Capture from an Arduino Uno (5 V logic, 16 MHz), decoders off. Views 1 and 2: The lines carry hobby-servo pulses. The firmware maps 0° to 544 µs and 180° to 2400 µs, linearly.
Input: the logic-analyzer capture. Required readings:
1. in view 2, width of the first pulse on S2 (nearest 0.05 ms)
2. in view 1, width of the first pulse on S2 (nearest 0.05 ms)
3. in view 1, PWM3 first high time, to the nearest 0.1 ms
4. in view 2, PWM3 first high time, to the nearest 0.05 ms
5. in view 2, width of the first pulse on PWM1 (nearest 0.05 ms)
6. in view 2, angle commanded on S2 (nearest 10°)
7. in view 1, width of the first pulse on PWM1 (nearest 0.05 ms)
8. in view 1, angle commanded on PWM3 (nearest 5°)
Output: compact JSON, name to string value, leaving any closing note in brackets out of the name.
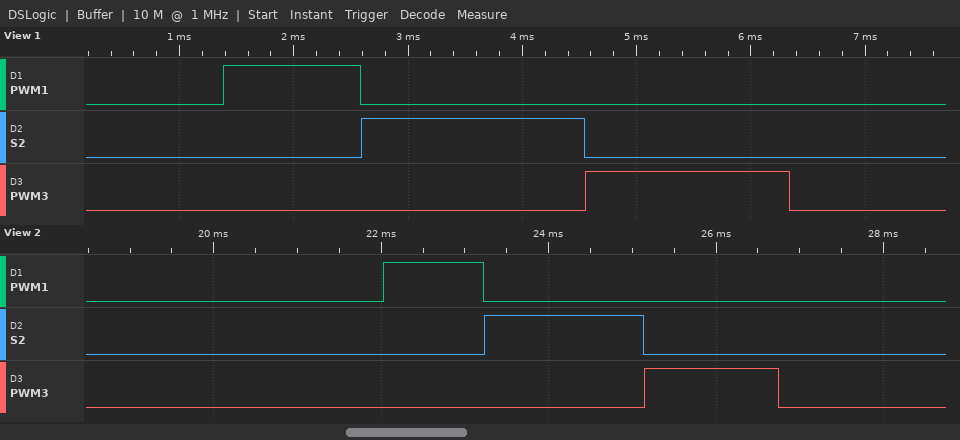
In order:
{"in view 2, width of the first pulse on S2": "1.90 ms", "in view 1, width of the first pulse on S2": "1.95 ms", "in view 1, PWM3 first high time, to the nearest 0.1 ms": "1.8 ms", "in view 2, PWM3 first high time, to the nearest 0.05 ms": "1.60 ms", "in view 2, width of the first pulse on PWM1": "1.20 ms", "in view 2, angle commanded on S2": "130°", "in view 1, width of the first pulse on PWM1": "1.20 ms", "in view 1, angle commanded on PWM3": "120°"}
